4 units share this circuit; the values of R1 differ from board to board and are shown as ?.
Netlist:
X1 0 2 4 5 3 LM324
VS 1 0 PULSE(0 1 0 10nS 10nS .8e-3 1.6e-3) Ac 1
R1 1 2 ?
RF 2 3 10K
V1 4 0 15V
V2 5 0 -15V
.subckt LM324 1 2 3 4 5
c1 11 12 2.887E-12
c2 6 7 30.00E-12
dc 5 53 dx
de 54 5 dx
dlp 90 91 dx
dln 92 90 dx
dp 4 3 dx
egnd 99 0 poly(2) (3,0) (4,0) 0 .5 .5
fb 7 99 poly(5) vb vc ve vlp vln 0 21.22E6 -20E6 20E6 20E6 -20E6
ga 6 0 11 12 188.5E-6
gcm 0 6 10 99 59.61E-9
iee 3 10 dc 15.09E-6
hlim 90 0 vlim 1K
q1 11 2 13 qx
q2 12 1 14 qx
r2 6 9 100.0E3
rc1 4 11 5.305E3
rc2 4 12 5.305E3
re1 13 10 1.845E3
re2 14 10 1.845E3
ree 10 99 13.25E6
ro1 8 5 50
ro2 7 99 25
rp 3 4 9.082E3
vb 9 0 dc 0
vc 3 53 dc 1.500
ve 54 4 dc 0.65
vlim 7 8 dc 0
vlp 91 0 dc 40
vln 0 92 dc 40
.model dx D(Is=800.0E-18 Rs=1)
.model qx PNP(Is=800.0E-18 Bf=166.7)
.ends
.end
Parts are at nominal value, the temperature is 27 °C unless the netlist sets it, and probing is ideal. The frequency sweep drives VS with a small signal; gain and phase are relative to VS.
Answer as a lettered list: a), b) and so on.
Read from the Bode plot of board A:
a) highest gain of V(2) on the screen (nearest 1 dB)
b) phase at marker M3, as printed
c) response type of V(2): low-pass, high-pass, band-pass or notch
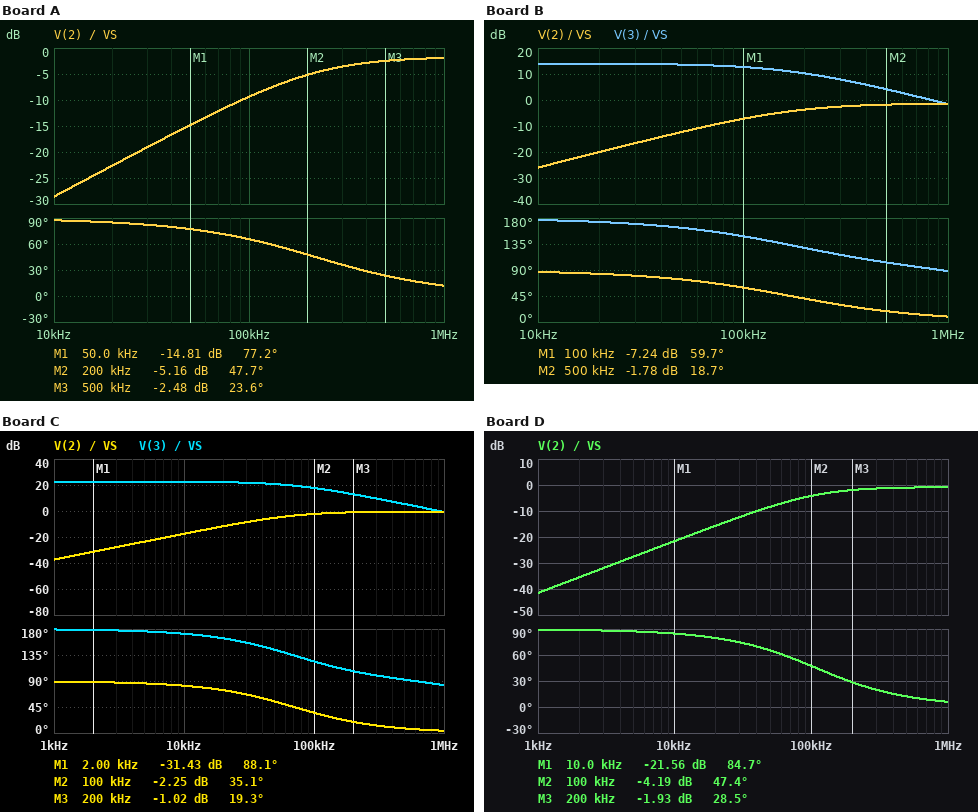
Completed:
a) -2 dB
b) 23.6 deg
c) high-pass
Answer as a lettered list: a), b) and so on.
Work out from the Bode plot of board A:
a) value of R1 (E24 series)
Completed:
a) 2.7 kΩ
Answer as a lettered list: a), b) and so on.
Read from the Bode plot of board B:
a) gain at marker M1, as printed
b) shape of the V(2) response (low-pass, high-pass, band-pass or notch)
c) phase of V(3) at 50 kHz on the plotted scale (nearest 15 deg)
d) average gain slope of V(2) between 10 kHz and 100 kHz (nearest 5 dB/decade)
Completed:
a) -7.24 dB
b) high-pass
c) 165 deg
d) 20 dB/decade
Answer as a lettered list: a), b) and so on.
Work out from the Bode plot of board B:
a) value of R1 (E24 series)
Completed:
a) 2 kΩ
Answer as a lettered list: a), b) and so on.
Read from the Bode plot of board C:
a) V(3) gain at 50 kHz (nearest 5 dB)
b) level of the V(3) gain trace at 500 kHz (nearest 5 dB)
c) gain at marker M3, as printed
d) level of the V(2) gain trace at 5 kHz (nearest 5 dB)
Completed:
a) 20 dB
b) 5 dB
c) -1.02 dB
d) -25 dB
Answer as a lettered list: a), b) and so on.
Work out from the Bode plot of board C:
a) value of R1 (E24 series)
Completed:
a) 750 Ω
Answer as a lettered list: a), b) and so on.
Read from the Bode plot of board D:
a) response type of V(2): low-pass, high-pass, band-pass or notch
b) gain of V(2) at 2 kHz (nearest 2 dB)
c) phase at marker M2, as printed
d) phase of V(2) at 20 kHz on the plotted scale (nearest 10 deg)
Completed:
a) high-pass
b) -36 dB
c) 47.4 deg
d) 80 deg
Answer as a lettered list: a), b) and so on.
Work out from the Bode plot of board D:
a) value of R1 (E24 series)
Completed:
a) 1.2 kΩ
